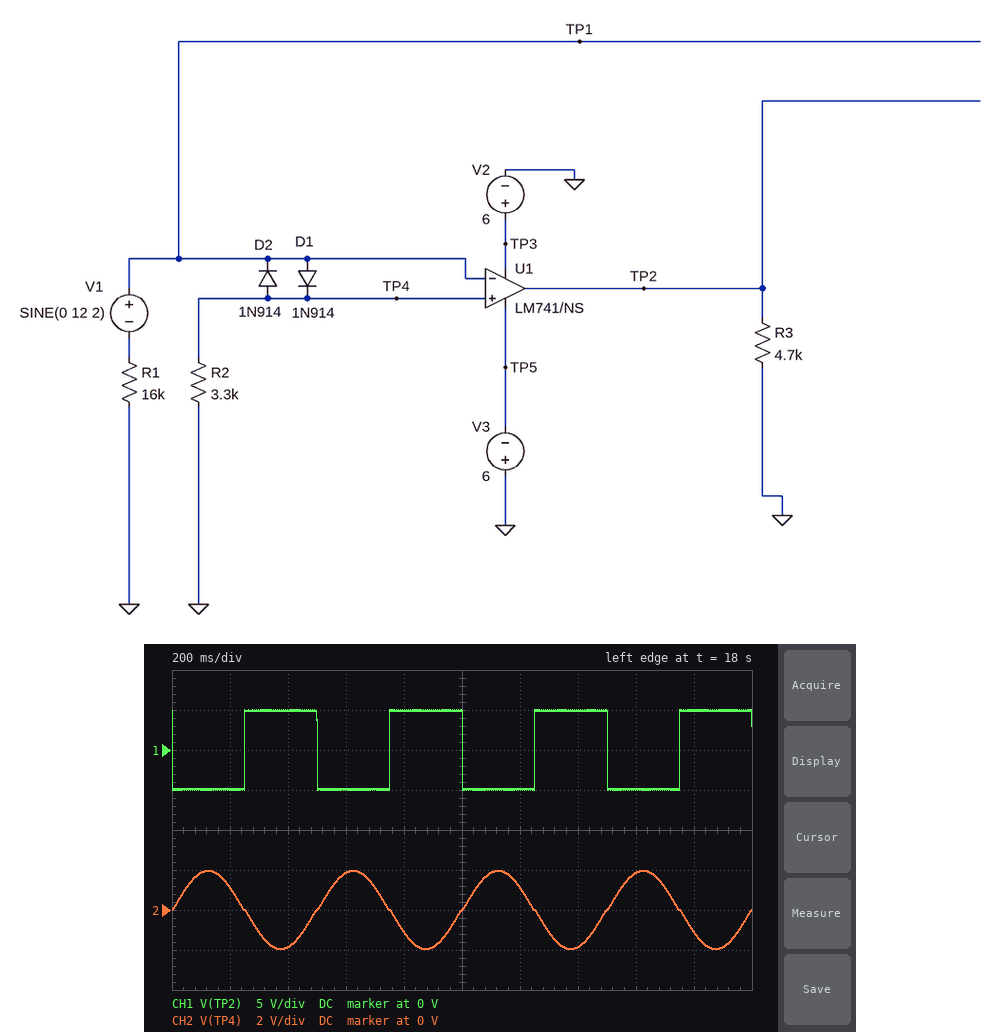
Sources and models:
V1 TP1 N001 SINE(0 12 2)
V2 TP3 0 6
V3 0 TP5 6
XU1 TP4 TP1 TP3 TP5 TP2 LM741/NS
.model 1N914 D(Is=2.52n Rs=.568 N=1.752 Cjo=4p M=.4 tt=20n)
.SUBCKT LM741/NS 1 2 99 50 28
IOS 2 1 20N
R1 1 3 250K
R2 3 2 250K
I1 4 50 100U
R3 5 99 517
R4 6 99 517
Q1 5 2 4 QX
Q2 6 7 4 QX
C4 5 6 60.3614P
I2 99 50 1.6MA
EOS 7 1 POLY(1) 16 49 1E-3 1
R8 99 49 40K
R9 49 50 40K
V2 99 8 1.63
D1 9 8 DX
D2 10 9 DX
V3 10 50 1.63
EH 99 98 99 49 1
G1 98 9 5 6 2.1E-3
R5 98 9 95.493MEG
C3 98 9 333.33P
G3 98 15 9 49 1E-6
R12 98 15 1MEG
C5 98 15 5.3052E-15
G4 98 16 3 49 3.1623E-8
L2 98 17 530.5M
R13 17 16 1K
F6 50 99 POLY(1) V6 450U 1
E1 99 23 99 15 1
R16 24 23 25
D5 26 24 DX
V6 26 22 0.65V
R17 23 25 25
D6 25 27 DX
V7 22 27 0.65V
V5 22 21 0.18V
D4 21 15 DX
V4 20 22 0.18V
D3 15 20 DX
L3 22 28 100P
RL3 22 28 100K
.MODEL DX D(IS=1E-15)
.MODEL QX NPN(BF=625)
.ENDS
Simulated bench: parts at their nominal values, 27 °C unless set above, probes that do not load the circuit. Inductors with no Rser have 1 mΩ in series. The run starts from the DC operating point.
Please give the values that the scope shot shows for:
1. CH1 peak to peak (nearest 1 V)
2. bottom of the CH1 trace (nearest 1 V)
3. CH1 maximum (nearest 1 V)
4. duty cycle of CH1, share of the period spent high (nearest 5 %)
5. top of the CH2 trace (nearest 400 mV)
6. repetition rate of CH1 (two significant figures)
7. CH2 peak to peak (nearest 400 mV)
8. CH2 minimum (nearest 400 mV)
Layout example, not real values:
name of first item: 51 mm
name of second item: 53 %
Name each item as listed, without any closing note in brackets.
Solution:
CH1 peak to peak: 10 V
bottom of the CH1 trace: -5 V
CH1 maximum: 5 V
duty cycle of CH1, share of the period spent high: 50 %
top of the CH2 trace: 2.0 V
repetition rate of CH1: 2.0 Hz
CH2 peak to peak: 4.0 V
CH2 minimum: -2.0 V
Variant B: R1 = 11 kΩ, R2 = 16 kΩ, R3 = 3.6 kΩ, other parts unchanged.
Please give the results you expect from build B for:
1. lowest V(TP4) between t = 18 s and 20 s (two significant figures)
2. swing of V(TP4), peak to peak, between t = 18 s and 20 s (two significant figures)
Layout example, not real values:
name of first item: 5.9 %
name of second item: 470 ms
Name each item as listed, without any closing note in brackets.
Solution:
lowest V(TP4) between t = 18 s and 20 s: -6.8 V
swing of V(TP4), peak to peak, between t = 18 s and 20 s: 13 V
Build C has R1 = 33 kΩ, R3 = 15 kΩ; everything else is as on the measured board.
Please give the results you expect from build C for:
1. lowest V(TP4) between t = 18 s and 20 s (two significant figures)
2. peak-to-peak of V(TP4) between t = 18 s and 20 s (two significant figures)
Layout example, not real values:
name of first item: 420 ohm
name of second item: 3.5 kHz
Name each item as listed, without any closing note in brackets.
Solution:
lowest V(TP4) between t = 18 s and 20 s: -1.0 V
peak-to-peak of V(TP4) between t = 18 s and 20 s: 2.1 V
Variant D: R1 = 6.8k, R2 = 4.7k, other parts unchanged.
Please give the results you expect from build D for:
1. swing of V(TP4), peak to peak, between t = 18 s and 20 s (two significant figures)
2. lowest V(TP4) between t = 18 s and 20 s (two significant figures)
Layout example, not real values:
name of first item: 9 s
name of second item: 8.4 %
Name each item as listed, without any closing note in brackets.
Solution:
swing of V(TP4), peak to peak, between t = 18 s and 20 s: 9.3 V
lowest V(TP4) between t = 18 s and 20 s: -4.7 V
